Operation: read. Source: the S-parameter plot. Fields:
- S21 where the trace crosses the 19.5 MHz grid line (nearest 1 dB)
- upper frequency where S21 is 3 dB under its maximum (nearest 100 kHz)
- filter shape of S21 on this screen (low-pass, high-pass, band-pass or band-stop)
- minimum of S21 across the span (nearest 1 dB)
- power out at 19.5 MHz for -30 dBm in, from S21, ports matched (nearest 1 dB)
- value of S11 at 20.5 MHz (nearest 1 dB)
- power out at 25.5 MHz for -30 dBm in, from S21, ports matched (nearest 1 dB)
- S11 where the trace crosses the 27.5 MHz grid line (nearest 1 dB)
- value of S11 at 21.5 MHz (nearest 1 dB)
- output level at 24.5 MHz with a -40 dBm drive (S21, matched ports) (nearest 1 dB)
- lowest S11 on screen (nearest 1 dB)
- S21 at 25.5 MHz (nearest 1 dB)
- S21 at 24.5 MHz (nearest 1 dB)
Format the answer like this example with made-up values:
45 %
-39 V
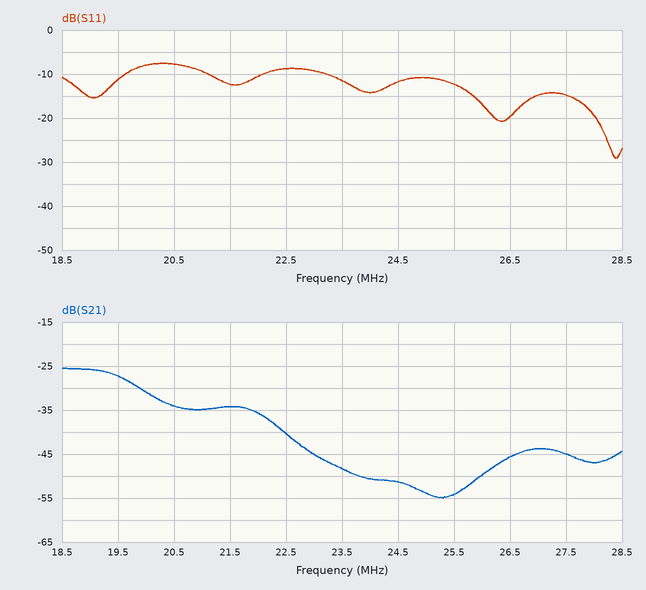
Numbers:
-27 dB
19.7 MHz
low-pass
-55 dB
-57 dBm
-8 dB
-84 dBm
-15 dB
-12 dB
-91 dBm
-29 dB
-54 dB
-51 dB
